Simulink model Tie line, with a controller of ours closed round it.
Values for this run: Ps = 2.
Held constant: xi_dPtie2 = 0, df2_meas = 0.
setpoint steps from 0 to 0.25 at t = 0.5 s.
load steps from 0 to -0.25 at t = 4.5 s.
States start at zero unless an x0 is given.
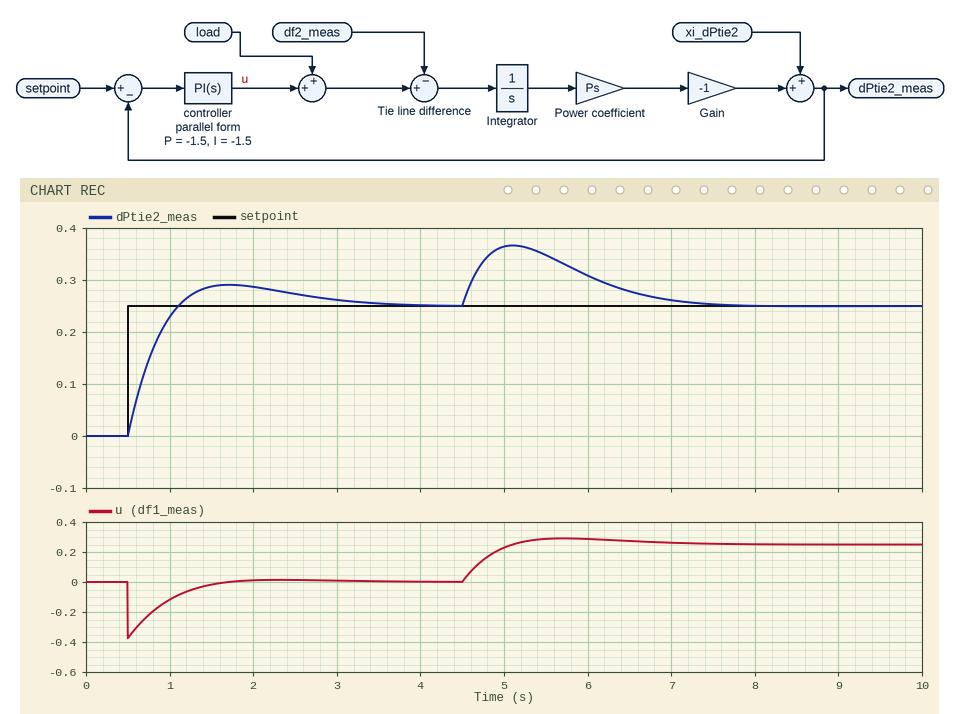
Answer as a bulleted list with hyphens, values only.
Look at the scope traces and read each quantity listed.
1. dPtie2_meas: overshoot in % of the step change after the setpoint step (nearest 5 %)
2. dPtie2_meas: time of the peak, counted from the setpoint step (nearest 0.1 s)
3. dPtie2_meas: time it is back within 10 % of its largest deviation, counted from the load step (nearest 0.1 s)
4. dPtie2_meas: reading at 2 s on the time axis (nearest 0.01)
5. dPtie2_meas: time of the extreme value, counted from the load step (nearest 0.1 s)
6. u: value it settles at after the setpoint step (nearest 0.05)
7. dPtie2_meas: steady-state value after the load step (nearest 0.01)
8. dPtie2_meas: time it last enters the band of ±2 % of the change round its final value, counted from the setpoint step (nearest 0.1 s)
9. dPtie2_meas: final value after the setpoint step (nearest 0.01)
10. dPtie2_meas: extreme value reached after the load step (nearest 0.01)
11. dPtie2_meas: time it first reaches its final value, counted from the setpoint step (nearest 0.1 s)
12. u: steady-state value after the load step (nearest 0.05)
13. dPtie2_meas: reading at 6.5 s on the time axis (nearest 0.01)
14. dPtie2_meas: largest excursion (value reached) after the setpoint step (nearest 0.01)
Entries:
- 15 %
- 1.2 s
- 2.5 s
- 0.29
- 0.6 s
- 0.00
- 0.25
- 3.0 s
- 0.25
- 0.37
- 0.6 s
- 0.25
- 0.28
- 0.29
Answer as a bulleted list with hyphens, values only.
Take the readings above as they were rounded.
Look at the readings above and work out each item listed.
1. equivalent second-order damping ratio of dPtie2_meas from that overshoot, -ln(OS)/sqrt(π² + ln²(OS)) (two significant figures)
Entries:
- 0.52
